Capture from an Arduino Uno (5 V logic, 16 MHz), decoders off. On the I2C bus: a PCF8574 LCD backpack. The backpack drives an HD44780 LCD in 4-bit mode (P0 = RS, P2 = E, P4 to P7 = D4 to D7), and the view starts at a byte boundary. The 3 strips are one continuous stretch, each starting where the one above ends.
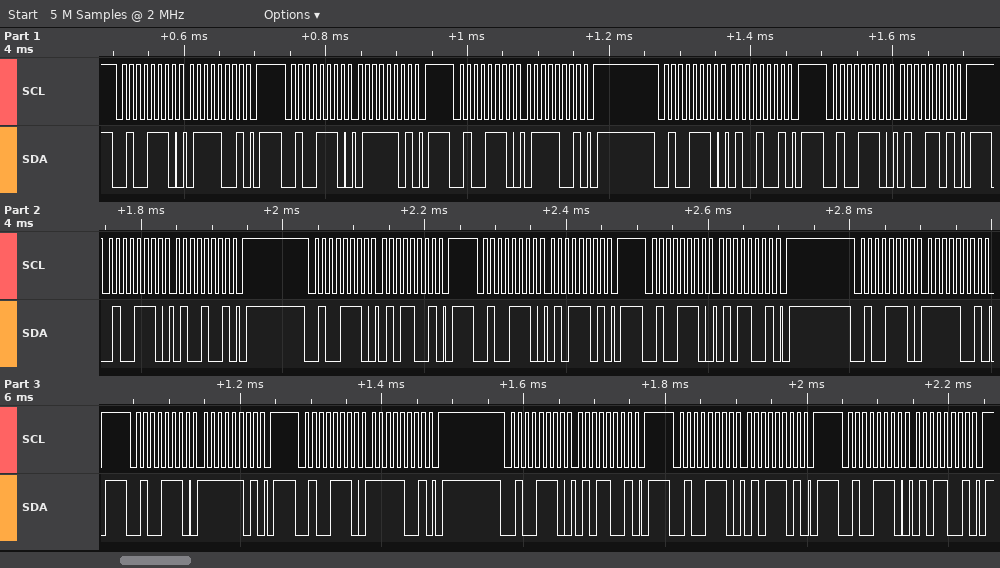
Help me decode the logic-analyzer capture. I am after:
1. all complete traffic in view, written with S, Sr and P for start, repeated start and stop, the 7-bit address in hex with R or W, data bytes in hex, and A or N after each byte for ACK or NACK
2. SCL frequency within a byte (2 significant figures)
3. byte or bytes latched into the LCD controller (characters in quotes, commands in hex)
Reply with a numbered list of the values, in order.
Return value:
1. S 27W A 79 A P S 27W A 7D A P S 27W A 79 A P S 27W A 49 A P S 27W A 4D A P S 27W A 49 A P S 27W A 59 A P S 27W A 5D A P S 27W A 59 A P S 27W A F9 A P S 27W A FD A P S 27W A F9 A P S 27W A 59 A P S 27W A 5D A P S 27W A 59 A P
2. 100 kHz
3. 't' '_'
